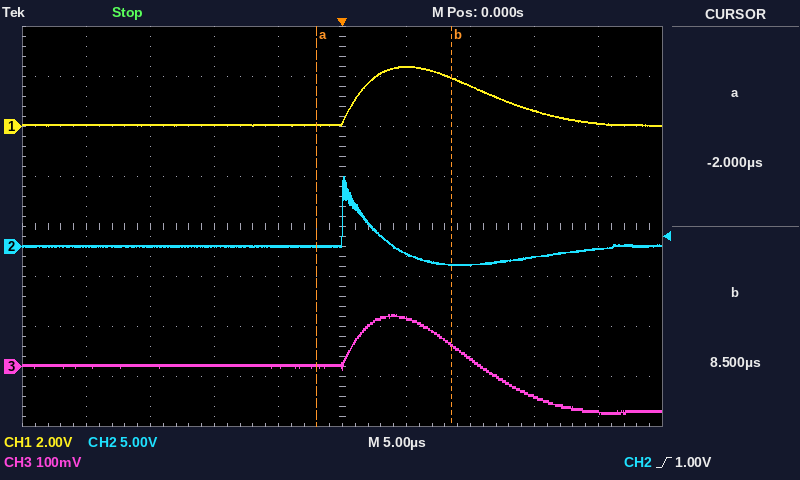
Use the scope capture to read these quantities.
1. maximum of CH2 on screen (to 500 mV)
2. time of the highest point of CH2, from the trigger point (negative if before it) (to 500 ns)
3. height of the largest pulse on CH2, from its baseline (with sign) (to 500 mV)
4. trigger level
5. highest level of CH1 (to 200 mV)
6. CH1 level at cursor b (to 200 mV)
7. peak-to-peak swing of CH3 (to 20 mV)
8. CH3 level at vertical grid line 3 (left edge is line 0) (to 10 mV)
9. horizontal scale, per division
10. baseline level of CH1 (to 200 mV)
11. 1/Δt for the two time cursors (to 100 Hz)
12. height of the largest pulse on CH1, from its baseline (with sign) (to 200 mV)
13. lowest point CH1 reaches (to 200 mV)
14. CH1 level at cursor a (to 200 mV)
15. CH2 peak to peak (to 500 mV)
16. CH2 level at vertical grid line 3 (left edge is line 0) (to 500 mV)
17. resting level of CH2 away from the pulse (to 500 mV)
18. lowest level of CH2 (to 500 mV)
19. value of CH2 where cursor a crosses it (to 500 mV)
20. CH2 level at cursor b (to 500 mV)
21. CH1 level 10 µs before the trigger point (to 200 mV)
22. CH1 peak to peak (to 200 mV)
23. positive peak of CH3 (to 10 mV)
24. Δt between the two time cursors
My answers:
7.0 V
0.0 µs
+7.0 V
1.00 V
2.4 V
2.0 V
200 mV
0 mV
5 µs
0.0 V
95.2 kHz
+2.4 V
0.0 V
0.0 V
9.0 V
0.0 V
0.0 V
-2.0 V
0.0 V
-2.0 V
0.0 V
2.4 V
100 mV
10.5 µs
